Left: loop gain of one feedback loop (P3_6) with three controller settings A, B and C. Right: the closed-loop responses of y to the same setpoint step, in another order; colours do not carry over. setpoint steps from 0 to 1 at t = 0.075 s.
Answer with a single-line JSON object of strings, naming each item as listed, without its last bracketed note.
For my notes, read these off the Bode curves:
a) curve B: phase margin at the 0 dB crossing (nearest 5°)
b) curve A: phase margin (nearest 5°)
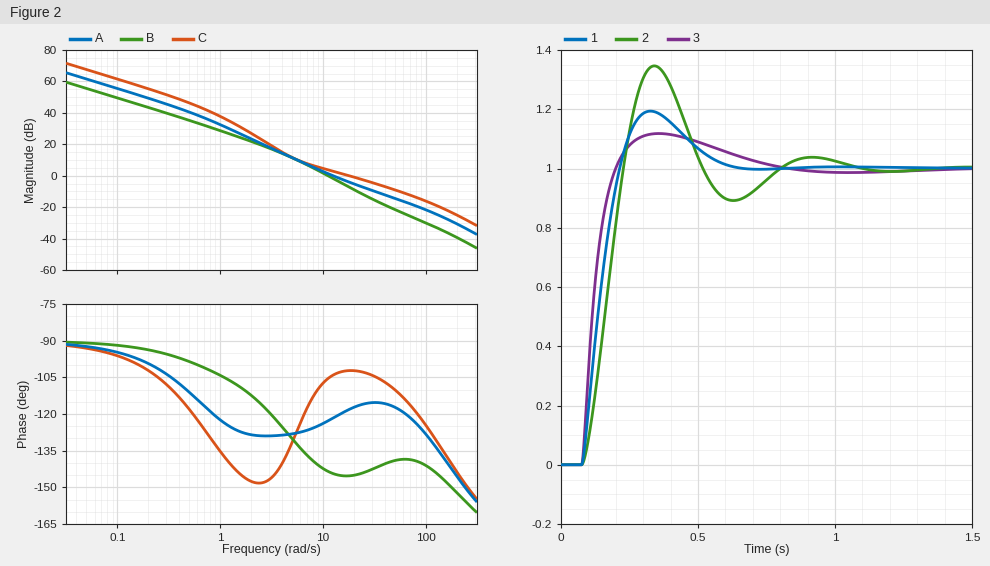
{"curve B: phase margin at the 0 dB crossing": "35°", "curve A: phase margin": "60°"}
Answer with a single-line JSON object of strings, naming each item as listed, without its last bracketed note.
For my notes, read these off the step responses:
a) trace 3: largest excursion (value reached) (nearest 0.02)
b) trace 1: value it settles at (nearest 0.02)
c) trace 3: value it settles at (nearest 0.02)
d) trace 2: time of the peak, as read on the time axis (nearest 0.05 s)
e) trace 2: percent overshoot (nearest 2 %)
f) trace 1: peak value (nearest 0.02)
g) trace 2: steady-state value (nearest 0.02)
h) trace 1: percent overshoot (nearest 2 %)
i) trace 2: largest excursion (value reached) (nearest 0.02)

{"trace 3: largest excursion (value reached)": "1.12", "trace 1: value it settles at": "1.00", "trace 3: value it settles at": "1.00", "trace 2: time of the peak, as read on the time axis": "0.35 s", "trace 2: percent overshoot": "34 %", "trace 1: peak value": "1.20", "trace 2: steady-state value": "1.00", "trace 1: percent overshoot": "20 %", "trace 2: largest excursion (value reached)": "1.34"}
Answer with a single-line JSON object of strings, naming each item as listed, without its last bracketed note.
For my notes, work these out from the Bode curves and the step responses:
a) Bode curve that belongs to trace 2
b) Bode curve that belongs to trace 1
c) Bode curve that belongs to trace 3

{"Bode curve that belongs to trace 2": "B", "Bode curve that belongs to trace 1": "A", "Bode curve that belongs to trace 3": "C"}
